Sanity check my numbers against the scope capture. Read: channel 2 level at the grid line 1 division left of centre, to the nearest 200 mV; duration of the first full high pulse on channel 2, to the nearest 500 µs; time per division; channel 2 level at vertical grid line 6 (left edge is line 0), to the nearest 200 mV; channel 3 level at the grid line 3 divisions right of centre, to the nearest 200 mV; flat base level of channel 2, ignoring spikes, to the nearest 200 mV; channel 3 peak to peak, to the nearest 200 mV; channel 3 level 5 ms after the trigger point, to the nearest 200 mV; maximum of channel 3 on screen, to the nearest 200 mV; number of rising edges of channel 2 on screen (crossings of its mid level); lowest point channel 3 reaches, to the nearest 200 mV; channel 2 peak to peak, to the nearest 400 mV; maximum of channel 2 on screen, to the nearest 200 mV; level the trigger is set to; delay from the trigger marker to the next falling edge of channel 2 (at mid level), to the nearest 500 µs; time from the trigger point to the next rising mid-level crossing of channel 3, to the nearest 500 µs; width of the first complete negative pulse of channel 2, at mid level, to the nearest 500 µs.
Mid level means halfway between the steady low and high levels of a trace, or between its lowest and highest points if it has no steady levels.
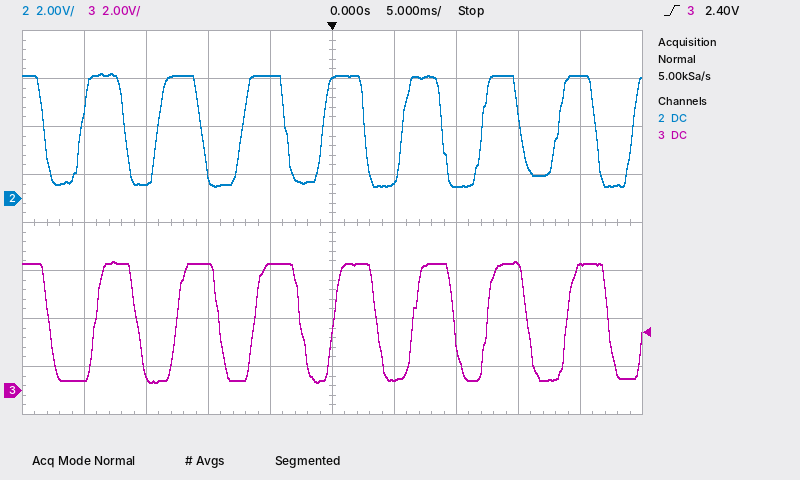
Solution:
5.2 V
3.5 ms
5 ms
800 mV
5.2 V
600 mV
5.0 V
400 mV
5.4 V
8
400 mV
4.8 V
5.2 V
2.40 V
2.5 ms
6.5 ms
3.0 ms
